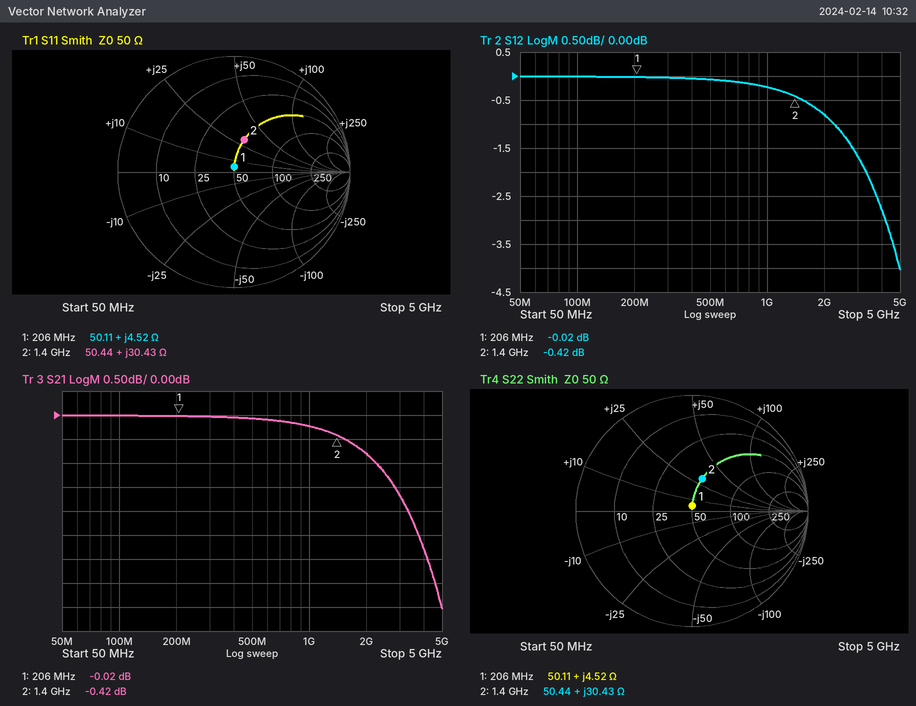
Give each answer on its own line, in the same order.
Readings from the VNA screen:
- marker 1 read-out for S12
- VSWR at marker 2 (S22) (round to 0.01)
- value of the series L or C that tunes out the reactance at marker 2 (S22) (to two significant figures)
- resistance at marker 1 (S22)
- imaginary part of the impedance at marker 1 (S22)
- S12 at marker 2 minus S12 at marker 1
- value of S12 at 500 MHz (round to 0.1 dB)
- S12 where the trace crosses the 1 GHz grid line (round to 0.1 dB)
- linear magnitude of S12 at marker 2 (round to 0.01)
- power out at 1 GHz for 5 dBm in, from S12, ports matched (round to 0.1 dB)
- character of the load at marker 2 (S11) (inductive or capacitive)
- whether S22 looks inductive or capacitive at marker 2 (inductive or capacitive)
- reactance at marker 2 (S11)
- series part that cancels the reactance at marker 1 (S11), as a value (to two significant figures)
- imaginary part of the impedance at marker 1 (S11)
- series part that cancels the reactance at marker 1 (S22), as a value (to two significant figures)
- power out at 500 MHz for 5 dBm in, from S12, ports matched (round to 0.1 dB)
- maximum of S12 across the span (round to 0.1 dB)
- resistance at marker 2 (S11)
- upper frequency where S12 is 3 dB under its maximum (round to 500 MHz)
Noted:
-0.02 dB
1.82
3.7 pF
50.11 Ω
+4.52 Ω
-0.40 dB
-0.1 dB
-0.2 dB
0.95
4.8 dBm
inductive
inductive
+30.43 Ω
170 pF
+4.52 Ω
170 pF
4.9 dBm
0.0 dB
50.44 Ω
4.0 GHz
